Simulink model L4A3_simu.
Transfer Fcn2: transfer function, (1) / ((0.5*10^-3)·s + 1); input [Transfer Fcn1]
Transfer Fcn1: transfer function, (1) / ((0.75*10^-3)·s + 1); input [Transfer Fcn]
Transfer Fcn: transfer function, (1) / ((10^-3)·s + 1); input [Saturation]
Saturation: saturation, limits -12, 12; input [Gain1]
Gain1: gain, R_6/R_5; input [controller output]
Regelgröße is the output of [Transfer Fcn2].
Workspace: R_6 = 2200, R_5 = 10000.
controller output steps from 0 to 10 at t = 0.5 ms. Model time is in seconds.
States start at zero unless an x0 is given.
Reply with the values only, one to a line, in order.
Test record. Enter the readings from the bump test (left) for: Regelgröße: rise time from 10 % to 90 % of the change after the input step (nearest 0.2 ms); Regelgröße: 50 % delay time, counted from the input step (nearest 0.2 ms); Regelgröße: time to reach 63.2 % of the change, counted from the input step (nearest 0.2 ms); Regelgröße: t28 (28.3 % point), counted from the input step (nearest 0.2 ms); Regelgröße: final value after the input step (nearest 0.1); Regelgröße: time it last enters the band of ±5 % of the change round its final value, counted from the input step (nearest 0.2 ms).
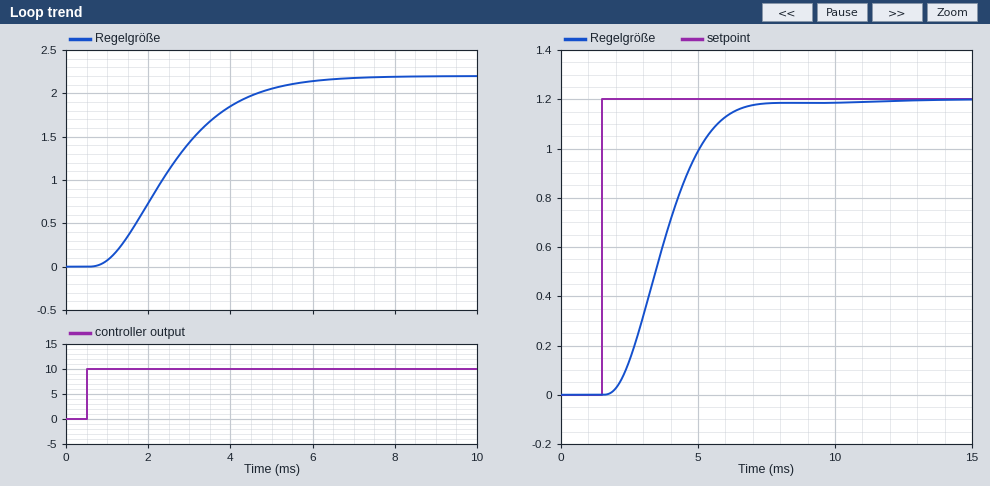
3.2 ms
2.0 ms
2.4 ms
1.4 ms
2.2
4.8 ms
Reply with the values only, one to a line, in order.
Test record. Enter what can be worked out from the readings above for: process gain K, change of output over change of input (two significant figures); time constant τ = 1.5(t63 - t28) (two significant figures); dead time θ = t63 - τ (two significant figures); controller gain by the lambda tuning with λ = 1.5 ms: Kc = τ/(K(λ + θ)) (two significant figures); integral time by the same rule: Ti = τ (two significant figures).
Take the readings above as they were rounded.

0.22
1.5 ms
0.90 ms
2.8
1.5 ms
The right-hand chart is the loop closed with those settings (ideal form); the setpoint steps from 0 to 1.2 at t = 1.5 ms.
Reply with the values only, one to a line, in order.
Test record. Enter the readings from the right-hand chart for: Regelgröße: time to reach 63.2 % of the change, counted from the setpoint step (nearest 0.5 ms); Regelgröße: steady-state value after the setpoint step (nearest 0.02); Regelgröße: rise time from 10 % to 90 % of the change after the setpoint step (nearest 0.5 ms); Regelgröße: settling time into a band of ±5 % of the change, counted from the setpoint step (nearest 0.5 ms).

2.5 ms
1.20
3.0 ms
4.5 ms
